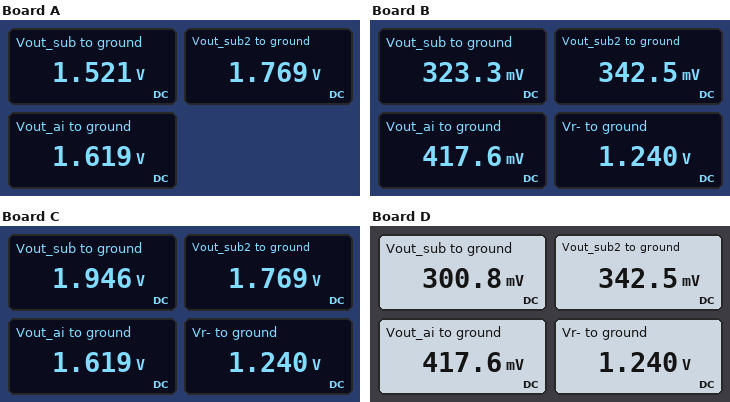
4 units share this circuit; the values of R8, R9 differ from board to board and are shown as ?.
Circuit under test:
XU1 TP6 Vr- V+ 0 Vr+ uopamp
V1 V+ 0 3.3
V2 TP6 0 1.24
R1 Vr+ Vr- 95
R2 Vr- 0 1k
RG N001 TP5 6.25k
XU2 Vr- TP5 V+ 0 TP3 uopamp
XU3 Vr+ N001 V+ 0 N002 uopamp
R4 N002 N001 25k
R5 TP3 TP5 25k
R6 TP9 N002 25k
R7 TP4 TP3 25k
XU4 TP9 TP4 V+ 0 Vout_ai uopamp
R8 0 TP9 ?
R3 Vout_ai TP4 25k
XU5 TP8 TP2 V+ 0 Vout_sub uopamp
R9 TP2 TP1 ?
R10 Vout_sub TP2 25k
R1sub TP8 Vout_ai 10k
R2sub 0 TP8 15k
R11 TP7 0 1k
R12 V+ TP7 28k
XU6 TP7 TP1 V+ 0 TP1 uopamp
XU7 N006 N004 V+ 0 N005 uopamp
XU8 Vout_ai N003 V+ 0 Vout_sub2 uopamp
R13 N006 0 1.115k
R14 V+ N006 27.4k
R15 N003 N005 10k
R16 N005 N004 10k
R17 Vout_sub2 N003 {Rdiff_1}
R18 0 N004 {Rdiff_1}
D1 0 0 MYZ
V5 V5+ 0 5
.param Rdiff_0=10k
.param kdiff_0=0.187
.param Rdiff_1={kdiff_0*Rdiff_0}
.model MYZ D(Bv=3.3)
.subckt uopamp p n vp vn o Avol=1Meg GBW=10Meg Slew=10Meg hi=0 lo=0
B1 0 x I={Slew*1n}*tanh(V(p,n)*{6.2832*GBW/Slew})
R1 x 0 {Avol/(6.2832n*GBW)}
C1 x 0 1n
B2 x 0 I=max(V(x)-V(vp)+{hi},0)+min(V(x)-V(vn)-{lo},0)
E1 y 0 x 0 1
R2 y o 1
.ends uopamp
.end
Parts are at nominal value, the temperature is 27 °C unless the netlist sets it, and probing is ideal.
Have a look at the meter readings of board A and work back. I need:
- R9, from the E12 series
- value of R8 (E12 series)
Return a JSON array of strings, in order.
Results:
["39 kΩ", "47 kΩ"]
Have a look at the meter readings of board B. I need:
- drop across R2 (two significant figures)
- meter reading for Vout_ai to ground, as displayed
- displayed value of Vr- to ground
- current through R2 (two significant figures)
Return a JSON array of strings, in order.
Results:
["1.2 V", "417.6 mV", "1.240 V", "1.2 mA"]
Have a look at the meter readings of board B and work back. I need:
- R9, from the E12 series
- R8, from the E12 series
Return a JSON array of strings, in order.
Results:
["47 kΩ", "12 kΩ"]
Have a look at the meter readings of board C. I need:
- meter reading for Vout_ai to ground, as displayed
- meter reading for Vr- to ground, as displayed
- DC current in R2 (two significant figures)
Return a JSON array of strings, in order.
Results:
["1.619 V", "1.240 V", "1.2 mA"]
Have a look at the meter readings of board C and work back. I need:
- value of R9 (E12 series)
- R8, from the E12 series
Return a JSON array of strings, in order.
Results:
["22 kΩ", "47 kΩ"]
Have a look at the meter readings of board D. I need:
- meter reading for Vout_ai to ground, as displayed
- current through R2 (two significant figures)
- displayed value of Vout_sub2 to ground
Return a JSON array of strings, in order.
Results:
["417.6 mV", "1.2 mA", "342.5 mV"]
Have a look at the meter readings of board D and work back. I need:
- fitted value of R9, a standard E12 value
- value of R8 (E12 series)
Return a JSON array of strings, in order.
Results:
["68 kΩ", "12 kΩ"]
